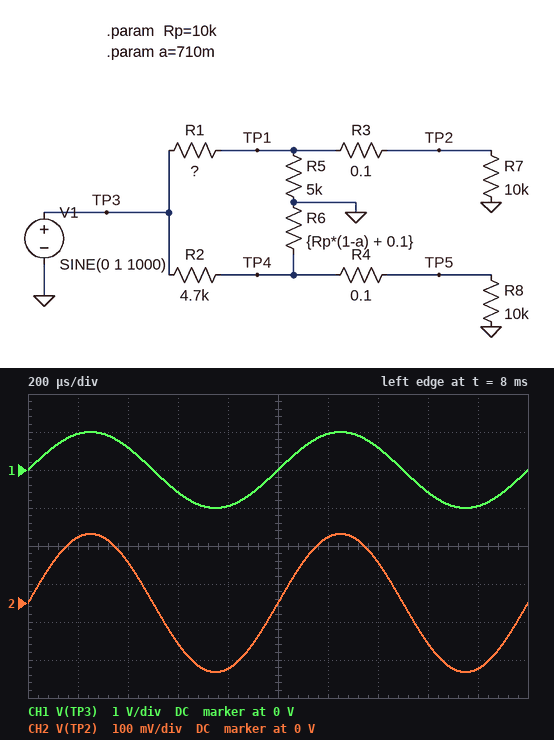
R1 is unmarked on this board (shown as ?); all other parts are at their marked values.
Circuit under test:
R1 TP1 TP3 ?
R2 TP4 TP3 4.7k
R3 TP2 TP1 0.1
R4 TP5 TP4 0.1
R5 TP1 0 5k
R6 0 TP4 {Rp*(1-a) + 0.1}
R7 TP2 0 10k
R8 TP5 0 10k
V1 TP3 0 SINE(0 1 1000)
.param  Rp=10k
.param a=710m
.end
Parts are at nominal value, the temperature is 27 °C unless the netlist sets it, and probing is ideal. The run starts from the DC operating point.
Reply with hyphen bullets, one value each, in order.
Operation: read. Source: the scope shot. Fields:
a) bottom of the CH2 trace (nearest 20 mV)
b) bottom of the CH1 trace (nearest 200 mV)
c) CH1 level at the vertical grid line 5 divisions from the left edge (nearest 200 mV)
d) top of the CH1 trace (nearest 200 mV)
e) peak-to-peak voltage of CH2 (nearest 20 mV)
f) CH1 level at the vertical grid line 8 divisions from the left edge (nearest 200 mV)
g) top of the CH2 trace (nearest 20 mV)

- -180 mV
- -1.0 V
- 0 V
- 1.0 V
- 360 mV
- -600 mV
- 180 mV
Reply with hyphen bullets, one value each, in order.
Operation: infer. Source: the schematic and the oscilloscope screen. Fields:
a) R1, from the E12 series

- 15 kΩ
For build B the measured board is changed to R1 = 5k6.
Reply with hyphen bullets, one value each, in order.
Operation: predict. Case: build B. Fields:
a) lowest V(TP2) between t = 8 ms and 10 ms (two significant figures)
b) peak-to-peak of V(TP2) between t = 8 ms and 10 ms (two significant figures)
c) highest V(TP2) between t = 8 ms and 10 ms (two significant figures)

- -370 mV
- 750 mV
- 370 mV
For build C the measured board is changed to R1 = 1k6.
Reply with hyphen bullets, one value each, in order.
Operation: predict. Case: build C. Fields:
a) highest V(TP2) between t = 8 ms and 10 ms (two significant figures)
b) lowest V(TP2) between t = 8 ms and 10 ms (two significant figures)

- 680 mV
- -680 mV
